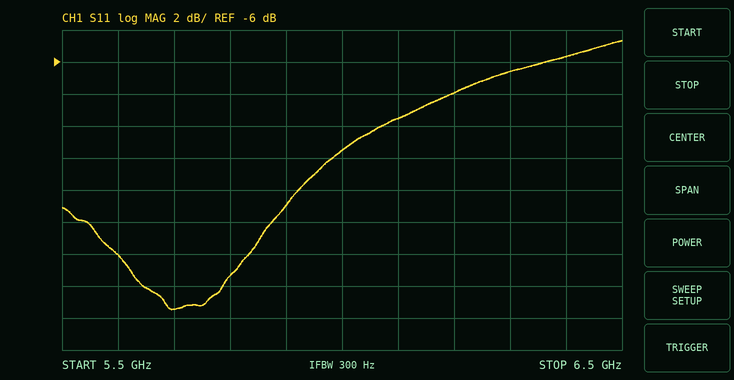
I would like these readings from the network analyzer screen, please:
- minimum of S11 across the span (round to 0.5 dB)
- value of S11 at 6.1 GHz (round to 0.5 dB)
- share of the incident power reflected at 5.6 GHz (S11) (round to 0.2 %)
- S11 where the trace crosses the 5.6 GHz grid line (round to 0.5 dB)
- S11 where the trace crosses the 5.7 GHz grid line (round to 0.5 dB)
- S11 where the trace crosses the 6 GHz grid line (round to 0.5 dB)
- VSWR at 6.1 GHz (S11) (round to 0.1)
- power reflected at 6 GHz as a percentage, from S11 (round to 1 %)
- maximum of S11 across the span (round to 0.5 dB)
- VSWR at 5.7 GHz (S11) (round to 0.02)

-21.5 dB
-9.5 dB
1.6 %
-18.0 dB
-21.5 dB
-11.5 dB
2.0
7 %
-4.5 dB
1.18
